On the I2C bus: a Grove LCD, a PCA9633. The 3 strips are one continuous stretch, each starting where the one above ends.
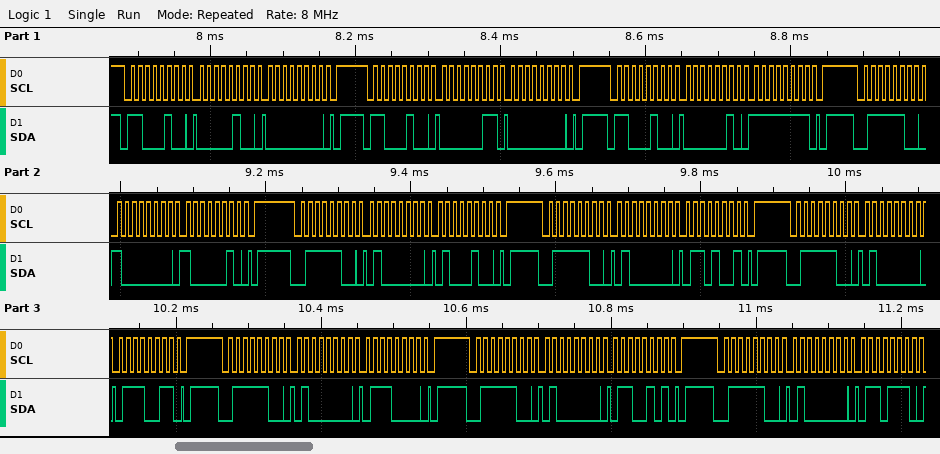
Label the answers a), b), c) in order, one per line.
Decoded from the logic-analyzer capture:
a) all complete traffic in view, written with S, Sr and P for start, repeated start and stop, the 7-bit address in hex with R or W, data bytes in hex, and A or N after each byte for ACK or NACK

a) S 62W A 04 A 00 A P S 62W A 03 A 00 A P S 62W A 02 A FF A P S 3EW A 80 A 82 A P S 3EW A 40 A 44 A P S 3EW A 40 A 69 A P S 3EW A 40 A 73 A P S 3EW A 40 A 70 A P S 3EW A 40 A 65 A P S 3EW A 40 A 6E A
